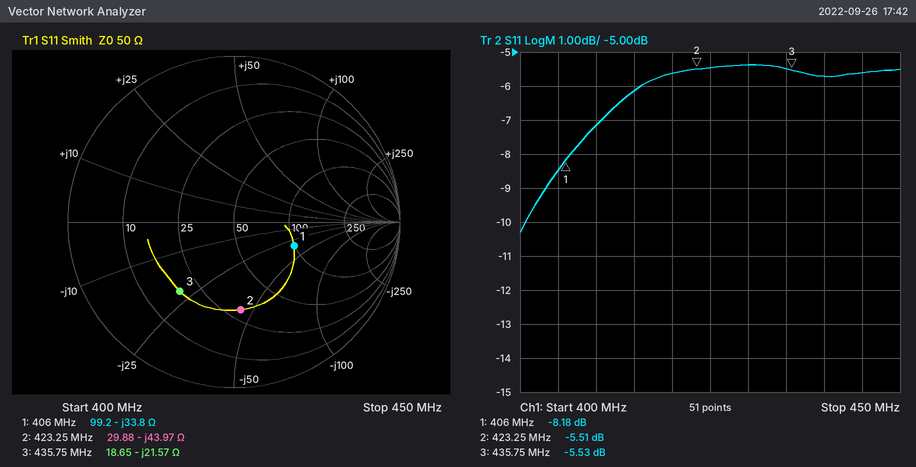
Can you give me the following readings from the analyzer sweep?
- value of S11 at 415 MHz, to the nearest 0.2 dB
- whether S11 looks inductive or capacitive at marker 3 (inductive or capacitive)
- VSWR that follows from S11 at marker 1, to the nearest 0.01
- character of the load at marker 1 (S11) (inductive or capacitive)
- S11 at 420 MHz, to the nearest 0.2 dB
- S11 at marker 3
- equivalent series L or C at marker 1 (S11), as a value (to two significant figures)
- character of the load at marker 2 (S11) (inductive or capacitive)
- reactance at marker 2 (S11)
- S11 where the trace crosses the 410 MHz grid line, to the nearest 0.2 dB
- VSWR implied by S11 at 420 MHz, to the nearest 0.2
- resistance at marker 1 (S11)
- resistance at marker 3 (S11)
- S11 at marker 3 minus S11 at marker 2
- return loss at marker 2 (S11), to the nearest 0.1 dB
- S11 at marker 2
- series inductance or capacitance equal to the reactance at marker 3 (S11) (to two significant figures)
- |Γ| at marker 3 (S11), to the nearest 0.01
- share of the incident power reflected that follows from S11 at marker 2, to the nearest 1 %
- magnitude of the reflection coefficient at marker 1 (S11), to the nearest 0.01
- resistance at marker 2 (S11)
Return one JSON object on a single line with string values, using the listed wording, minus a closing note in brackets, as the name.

{"value of S11 at 415 MHz, to the nearest 0.2 dB": "-6.2 dB", "whether S11 looks inductive or capacitive at marker 3": "capacitive", "VSWR that follows from S11 at marker 1, to the nearest 0.01": "2.28", "character of the load at marker 1 (S11)": "capacitive", "S11 at 420 MHz, to the nearest 0.2 dB": "-5.6 dB", "S11 at marker 3": "-5.53 dB", "equivalent series L or C at marker 1 (S11), as a value": "12 pF", "character of the load at marker 2 (S11)": "capacitive", "reactance at marker 2": "-43.97 Ω", "S11 where the trace crosses the 410 MHz grid line, to the nearest 0.2 dB": "-7.2 dB", "VSWR implied by S11 at 420 MHz, to the nearest 0.2": "3.2", "resistance at marker 1": "99.2 Ω", "resistance at marker 3": "18.65 Ω", "S11 at marker 3 minus S11 at marker 2": "-0.02 dB", "return loss at marker 2 (S11), to the nearest 0.1 dB": "5.5 dB", "S11 at marker 2": "-5.51 dB", "series inductance or capacitance equal to the reactance at marker 3 (S11)": "17 pF", "|Γ| at marker 3 (S11), to the nearest 0.01": "0.53", "share of the incident power reflected that follows from S11 at marker 2, to the nearest 1 %": "28 %", "magnitude of the reflection coefficient at marker 1 (S11), to the nearest 0.01": "0.39", "resistance at marker 2": "29.88 Ω"}
